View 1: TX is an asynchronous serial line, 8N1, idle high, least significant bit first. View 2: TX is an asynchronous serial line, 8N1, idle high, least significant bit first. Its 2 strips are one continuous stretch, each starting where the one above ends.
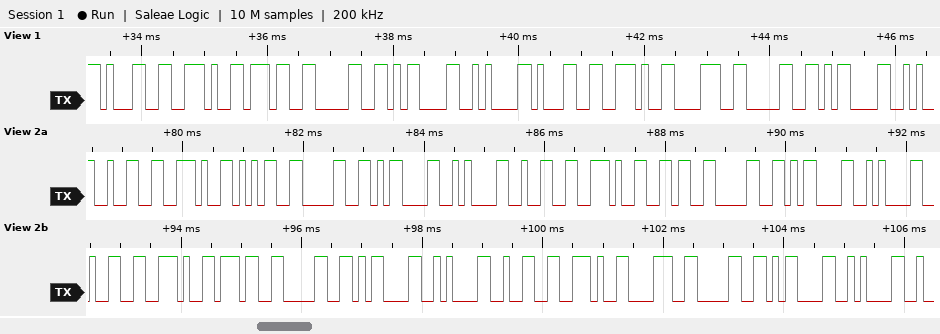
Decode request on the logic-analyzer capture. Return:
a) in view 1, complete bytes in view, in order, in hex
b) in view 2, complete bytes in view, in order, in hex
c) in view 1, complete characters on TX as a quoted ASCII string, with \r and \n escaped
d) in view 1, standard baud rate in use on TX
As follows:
31 2E 37 30 0D 0A 31 2E 38 30 0D
32 2E 35 30 0D 0A 32 2E 36 30 0D 0A 32 2E 37 30 0D 0A 32 2E 38 30 0D 0A
"1.70\r\n1.80\r"
9600 baud
